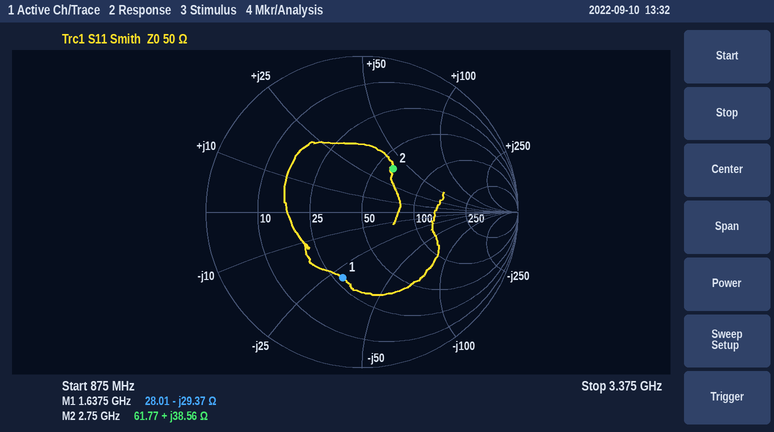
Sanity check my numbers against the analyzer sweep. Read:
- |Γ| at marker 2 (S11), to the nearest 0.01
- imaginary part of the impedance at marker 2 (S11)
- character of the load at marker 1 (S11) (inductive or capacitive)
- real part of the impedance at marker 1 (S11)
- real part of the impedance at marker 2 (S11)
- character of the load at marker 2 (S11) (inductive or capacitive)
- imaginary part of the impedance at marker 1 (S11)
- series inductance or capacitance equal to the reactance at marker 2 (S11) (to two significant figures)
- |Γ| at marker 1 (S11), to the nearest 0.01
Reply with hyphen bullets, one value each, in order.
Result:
- 0.34
- +38.56 Ω
- capacitive
- 28.01 Ω
- 61.77 Ω
- inductive
- -29.37 Ω
- 2.2 nH
- 0.44
